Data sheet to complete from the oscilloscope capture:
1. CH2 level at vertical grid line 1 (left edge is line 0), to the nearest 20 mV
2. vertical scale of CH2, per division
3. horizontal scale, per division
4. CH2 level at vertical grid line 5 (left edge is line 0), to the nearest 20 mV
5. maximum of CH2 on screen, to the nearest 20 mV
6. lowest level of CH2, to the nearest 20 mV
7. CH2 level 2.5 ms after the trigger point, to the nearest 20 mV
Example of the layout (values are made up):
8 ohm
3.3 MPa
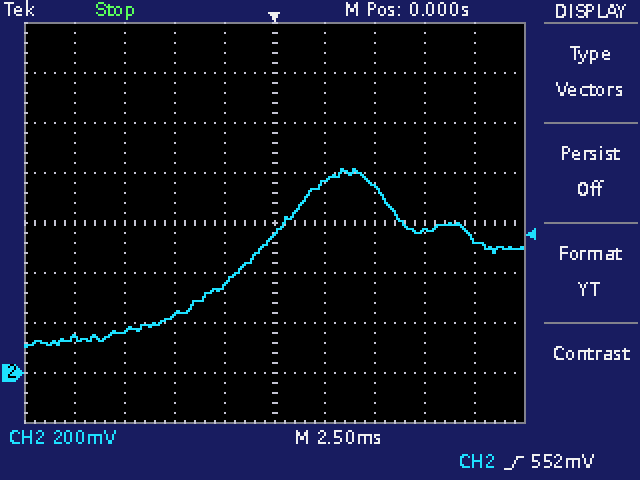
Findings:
140 mV
200 mV
2.5 ms
560 mV
820 mV
100 mV
760 mV
